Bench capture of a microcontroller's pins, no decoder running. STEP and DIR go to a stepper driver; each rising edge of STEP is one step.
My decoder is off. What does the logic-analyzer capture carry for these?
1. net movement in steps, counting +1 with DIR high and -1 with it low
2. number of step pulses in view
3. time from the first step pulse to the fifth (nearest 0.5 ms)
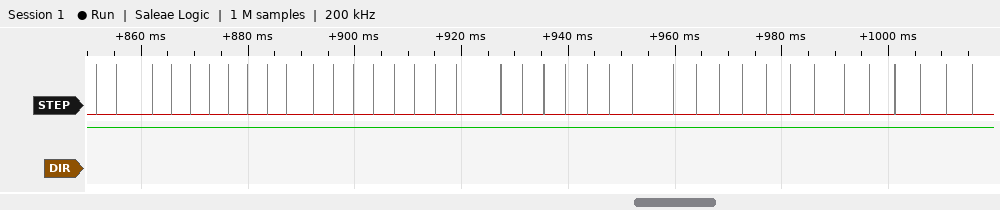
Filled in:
+38
38
17.5 ms
